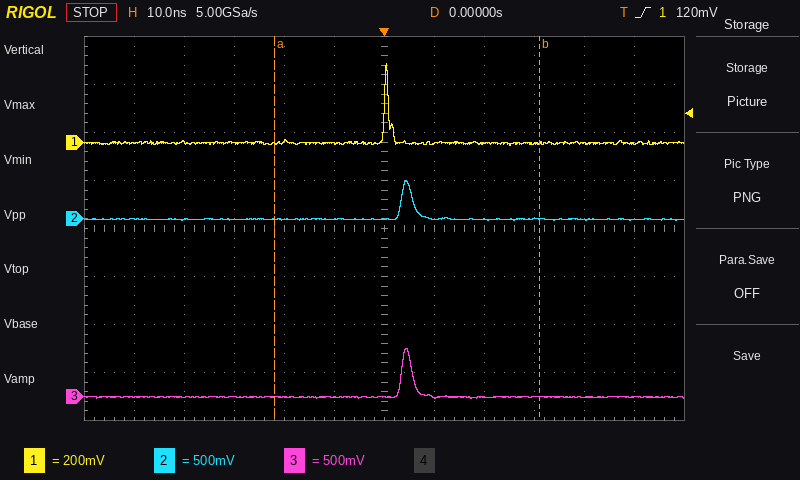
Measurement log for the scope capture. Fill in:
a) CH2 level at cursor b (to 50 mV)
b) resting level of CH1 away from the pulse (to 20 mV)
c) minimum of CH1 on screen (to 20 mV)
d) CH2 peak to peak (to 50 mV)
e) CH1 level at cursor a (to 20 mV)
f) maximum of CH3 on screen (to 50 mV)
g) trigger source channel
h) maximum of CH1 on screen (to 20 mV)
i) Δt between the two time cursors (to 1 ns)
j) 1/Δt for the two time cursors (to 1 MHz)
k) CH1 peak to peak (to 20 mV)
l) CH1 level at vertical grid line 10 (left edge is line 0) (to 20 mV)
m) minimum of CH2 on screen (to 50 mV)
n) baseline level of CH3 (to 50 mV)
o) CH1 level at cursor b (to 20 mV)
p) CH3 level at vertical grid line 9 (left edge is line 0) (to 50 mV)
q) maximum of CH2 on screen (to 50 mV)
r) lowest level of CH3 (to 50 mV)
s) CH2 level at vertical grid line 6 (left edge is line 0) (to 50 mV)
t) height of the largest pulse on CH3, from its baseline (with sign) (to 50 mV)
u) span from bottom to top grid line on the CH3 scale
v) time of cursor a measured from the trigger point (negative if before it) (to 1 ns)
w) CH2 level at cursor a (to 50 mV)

0 mV
0 mV
-20 mV
400 mV
0 mV
500 mV
CH1
320 mV
53 ns
19 MHz
340 mV
0 mV
0 mV
0 mV
0 mV
0 mV
400 mV
0 mV
0 mV
+500 mV
4 V
-22 ns
0 mV
